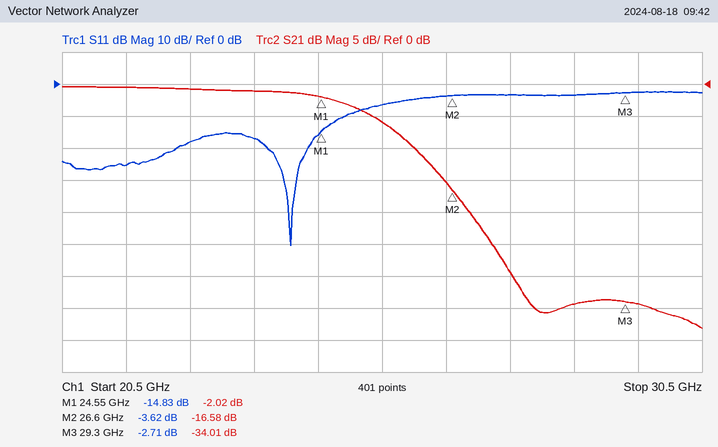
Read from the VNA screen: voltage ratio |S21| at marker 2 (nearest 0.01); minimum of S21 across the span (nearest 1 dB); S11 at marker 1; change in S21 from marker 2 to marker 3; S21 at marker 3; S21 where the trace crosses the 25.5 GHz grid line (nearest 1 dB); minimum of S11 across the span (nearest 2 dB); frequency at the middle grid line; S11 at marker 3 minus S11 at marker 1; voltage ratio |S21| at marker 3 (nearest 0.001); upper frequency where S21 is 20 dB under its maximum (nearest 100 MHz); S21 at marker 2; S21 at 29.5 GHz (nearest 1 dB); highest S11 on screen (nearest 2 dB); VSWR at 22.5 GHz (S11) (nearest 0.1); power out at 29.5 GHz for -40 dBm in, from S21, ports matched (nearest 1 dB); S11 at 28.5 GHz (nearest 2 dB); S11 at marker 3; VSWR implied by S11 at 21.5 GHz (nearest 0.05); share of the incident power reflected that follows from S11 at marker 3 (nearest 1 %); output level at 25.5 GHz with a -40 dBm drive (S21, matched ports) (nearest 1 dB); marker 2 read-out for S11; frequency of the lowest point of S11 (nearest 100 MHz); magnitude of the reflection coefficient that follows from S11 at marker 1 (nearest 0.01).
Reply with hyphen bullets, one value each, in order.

- 0.15
- -38 dB
- -14.83 dB
- -17.43 dB
- -34.01 dB
- -6 dB
- -50 dB
- 25.5 GHz
- 12.12 dB
- 0.020
- 26.9 GHz
- -16.58 dB
- -34 dB
- -2 dB
- 1.3
- -74 dBm
- -4 dB
- -2.71 dB
- 1.10
- 54 %
- -46 dBm
- -3.62 dB
- 24.1 GHz
- 0.18
